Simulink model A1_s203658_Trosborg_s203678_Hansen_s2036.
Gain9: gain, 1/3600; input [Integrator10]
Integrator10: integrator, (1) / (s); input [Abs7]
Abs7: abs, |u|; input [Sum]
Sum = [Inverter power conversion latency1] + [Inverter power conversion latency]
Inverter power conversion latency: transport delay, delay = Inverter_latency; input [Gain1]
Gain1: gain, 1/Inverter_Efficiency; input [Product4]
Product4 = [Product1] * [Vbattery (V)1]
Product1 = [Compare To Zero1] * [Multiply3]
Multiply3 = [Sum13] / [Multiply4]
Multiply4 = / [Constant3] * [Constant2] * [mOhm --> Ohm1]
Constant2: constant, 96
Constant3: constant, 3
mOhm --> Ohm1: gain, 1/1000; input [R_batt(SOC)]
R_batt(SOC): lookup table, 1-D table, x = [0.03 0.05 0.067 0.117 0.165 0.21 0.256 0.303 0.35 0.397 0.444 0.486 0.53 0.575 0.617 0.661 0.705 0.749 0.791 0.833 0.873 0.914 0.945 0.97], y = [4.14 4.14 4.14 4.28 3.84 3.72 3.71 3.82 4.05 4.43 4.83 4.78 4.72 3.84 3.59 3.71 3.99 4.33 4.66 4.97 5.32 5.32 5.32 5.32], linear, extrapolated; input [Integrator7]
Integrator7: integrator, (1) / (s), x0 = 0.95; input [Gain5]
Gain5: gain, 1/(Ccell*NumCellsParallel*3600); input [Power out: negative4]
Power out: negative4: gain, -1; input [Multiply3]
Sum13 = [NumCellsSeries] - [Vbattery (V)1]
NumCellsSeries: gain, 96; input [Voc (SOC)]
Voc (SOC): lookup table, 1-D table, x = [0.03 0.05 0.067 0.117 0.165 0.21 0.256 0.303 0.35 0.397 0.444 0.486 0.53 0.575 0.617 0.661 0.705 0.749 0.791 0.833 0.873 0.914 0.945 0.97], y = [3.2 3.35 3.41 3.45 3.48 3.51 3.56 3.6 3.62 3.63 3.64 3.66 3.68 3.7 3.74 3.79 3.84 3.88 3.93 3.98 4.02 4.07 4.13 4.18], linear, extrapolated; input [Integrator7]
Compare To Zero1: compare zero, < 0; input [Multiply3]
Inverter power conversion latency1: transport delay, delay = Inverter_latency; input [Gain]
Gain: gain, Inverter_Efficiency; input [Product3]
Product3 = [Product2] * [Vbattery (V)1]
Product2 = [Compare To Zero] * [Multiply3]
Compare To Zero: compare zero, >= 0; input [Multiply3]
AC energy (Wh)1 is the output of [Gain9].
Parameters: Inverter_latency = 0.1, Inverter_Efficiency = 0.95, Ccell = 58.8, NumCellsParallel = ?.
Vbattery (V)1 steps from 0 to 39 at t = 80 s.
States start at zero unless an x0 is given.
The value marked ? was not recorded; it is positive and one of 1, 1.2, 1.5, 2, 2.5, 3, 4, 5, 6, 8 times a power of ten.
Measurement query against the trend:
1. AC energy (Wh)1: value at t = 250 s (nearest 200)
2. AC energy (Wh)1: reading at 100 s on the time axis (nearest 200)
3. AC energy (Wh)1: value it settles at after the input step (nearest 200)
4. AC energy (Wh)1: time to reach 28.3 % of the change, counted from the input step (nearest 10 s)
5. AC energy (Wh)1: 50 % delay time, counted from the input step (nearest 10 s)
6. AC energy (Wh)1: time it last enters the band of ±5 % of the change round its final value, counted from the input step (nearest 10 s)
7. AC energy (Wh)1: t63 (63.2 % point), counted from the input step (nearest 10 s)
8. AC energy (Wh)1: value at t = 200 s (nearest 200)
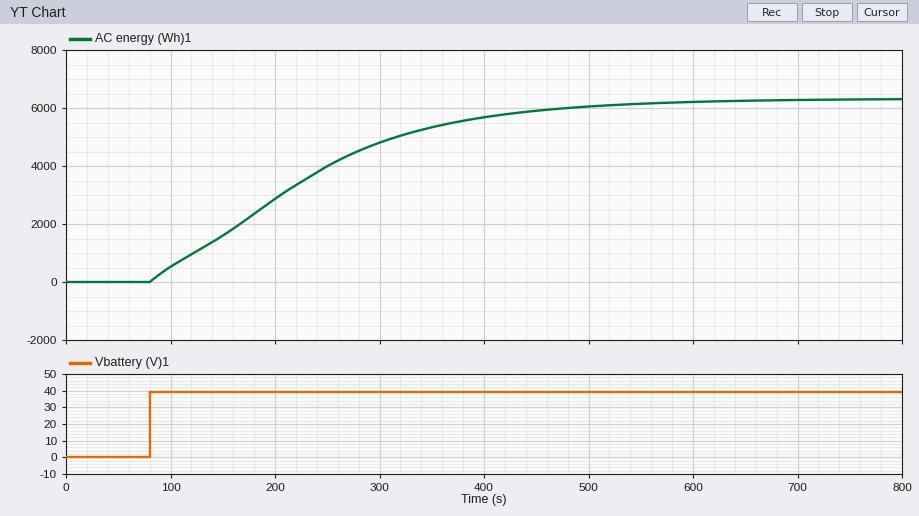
4000
600
6400
80 s
130 s
400 s
170 s
2800
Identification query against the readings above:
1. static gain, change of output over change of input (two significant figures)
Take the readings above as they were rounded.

160
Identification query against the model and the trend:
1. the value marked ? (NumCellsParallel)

3
